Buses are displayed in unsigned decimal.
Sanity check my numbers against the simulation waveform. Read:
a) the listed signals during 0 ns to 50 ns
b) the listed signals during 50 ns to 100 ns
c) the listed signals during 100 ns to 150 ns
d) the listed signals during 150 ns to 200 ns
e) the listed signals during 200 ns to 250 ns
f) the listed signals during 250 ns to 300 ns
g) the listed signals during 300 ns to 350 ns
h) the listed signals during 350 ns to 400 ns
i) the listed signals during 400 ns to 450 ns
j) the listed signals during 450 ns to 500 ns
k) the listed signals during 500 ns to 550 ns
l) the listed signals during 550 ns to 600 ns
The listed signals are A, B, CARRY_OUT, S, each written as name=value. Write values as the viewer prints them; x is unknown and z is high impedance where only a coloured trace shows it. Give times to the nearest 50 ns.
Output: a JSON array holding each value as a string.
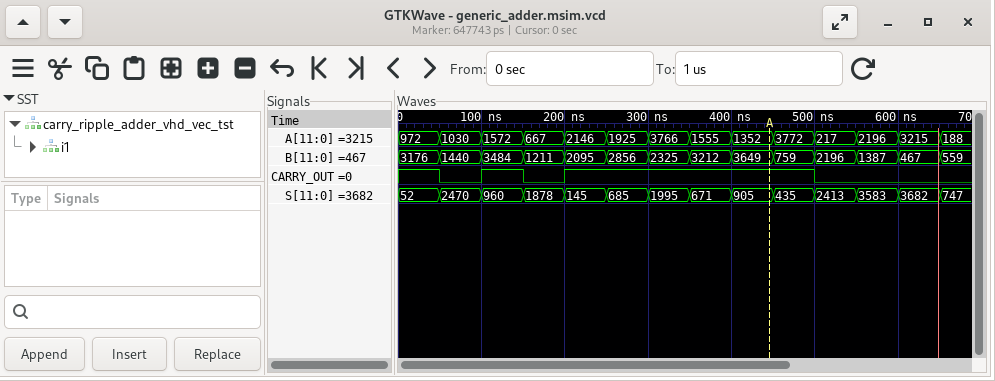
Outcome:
["A=972, B=3176, CARRY_OUT=1, S=52", "A=1030, B=1440, CARRY_OUT=0, S=2470", "A=1572, B=3484, CARRY_OUT=1, S=960", "A=667, B=1211, CARRY_OUT=0, S=1878", "A=2146, B=2095, CARRY_OUT=1, S=145", "A=1925, B=2856, CARRY_OUT=1, S=685", "A=3766, B=2325, CARRY_OUT=1, S=1995", "A=1555, B=3212, CARRY_OUT=1, S=671", "A=1352, B=3649, CARRY_OUT=1, S=905", "A=3772, B=759, CARRY_OUT=1, S=435", "A=217, B=2196, CARRY_OUT=0, S=2413", "A=2196, B=1387, CARRY_OUT=0, S=3583"]
